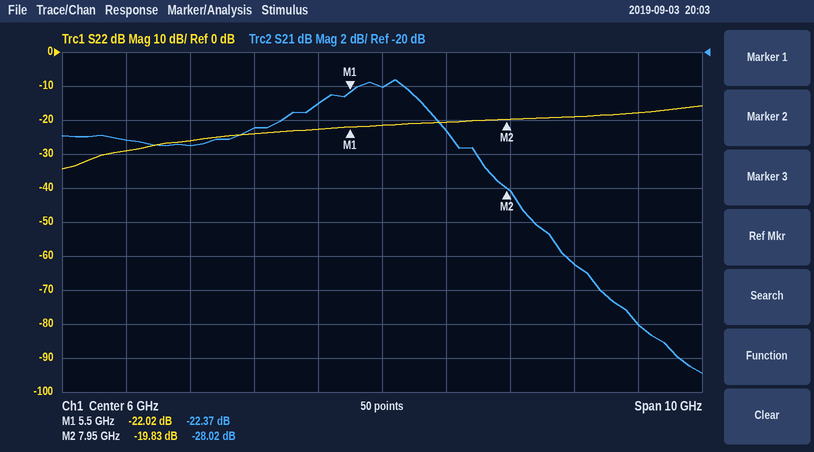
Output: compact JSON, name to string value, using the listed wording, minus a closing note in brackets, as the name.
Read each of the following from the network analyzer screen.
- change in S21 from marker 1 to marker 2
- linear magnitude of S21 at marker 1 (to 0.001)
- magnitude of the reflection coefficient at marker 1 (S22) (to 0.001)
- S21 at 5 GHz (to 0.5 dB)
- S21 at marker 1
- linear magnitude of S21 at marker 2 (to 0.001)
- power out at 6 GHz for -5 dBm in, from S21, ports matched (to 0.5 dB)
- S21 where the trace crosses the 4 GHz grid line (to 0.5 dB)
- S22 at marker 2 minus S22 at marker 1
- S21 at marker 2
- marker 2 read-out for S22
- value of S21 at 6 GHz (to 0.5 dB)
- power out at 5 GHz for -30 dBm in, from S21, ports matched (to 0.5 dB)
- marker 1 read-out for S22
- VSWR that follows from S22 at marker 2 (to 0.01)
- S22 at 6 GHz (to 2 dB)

{"change in S21 from marker 1 to marker 2": "-5.65 dB", "linear magnitude of S21 at marker 1": "0.076", "magnitude of the reflection coefficient at marker 1 (S22)": "0.079", "S21 at 5 GHz": "-23.0 dB", "S21 at marker 1": "-22.37 dB", "linear magnitude of S21 at marker 2": "0.040", "power out at 6 GHz for -5 dBm in, from S21, ports matched": "-27.0 dBm", "S21 where the trace crosses the 4 GHz grid line": "-24.5 dB", "S22 at marker 2 minus S22 at marker 1": "2.19 dB", "S21 at marker 2": "-28.02 dB", "marker 2 read-out for S22": "-19.83 dB", "value of S21 at 6 GHz": "-22.0 dB", "power out at 5 GHz for -30 dBm in, from S21, ports matched": "-53.0 dBm", "marker 1 read-out for S22": "-22.02 dB", "VSWR that follows from S22 at marker 2": "1.23", "S22 at 6 GHz": "-22 dB"}
